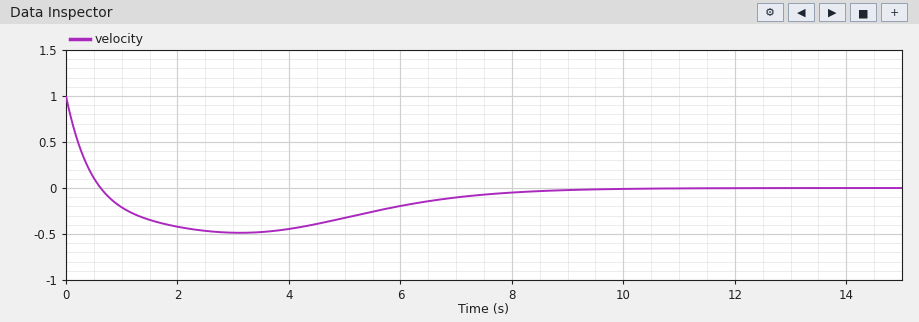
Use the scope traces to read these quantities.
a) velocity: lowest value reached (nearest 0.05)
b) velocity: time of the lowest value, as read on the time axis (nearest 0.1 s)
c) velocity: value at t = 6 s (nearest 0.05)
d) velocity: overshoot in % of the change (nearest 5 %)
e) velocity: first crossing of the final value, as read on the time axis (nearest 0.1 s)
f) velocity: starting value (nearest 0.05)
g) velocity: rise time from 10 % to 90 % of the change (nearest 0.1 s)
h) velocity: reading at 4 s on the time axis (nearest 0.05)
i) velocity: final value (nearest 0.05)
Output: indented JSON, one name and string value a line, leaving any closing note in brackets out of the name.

{
  "velocity: lowest value reached": "-0.50",
  "velocity: time of the lowest value, as read on the time axis": "3.1 s",
  "velocity: value at t = 6 s": "-0.20",
  "velocity: overshoot in % of the change": "50 %",
  "velocity: first crossing of the final value, as read on the time axis": "0.6 s",
  "velocity: starting value": "1.00",
  "velocity: rise time from 10 % to 90 % of the change": "0.5 s",
  "velocity: reading at 4 s on the time axis": "-0.45",
  "velocity: final value": "0.00"
}
